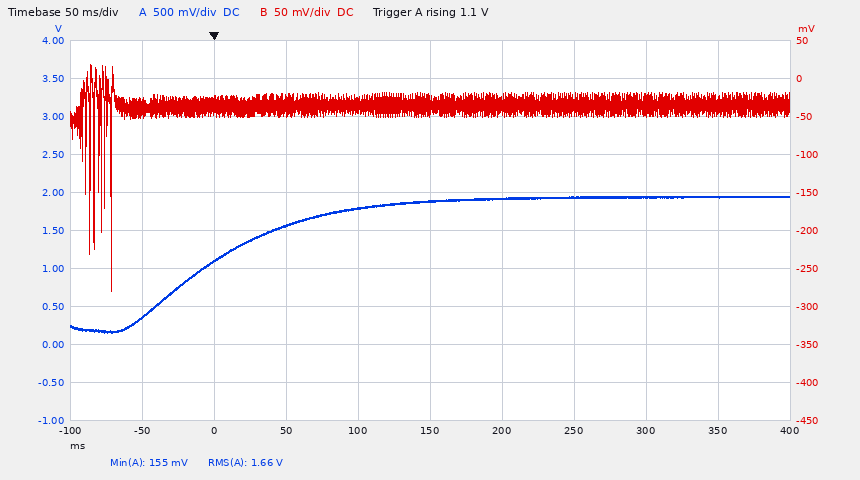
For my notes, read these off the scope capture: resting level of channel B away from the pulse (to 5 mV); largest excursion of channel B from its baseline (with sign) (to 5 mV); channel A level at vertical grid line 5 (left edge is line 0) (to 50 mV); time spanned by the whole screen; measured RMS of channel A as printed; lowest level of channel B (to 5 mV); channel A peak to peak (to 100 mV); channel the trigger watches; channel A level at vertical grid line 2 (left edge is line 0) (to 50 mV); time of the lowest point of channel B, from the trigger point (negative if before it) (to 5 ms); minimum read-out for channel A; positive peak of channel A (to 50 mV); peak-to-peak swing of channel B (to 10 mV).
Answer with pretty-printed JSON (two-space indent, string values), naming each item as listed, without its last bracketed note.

{
  "resting level of channel B away from the pulse": "-35 mV",
  "largest excursion of channel B from its baseline (with sign)": "-245 mV",
  "channel A level at vertical grid line 5 (left edge is line 0)": "1.90 V",
  "time spanned by the whole screen": "500 ms",
  "measured RMS of channel A as printed": "1.66 V",
  "lowest level of channel B": "-280 mV",
  "channel A peak to peak": "1.80 V",
  "channel the trigger watches": "channel A",
  "channel A level at vertical grid line 2 (left edge is line 0)": "1.10 V",
  "time of the lowest point of channel B, from the trigger point (negative if before it)": "-70 ms",
  "minimum read-out for channel A": "155 mV",
  "positive peak of channel A": "1.95 V",
  "peak-to-peak swing of channel B": "300 mV"
}
